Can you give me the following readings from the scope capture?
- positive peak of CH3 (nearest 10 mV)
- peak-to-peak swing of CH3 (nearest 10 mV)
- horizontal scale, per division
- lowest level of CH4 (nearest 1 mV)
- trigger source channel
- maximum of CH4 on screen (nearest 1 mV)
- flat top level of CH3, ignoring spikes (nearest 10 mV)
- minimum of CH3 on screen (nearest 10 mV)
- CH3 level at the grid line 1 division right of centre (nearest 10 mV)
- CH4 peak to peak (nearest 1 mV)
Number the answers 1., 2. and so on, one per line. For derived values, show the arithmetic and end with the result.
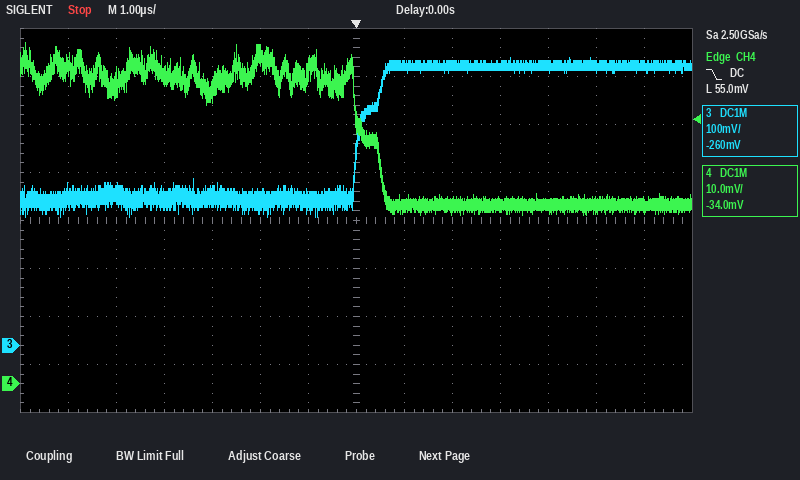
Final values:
1. 600 mV
2. 600 mV − (270 mV) = 330 mV
3. 1 µs
4. 35 mV
5. CH4
6. 71 mV
7. 580 mV
8. 270 mV
9. 580 mV
10. 71 mV − (35 mV) = 36 mV
